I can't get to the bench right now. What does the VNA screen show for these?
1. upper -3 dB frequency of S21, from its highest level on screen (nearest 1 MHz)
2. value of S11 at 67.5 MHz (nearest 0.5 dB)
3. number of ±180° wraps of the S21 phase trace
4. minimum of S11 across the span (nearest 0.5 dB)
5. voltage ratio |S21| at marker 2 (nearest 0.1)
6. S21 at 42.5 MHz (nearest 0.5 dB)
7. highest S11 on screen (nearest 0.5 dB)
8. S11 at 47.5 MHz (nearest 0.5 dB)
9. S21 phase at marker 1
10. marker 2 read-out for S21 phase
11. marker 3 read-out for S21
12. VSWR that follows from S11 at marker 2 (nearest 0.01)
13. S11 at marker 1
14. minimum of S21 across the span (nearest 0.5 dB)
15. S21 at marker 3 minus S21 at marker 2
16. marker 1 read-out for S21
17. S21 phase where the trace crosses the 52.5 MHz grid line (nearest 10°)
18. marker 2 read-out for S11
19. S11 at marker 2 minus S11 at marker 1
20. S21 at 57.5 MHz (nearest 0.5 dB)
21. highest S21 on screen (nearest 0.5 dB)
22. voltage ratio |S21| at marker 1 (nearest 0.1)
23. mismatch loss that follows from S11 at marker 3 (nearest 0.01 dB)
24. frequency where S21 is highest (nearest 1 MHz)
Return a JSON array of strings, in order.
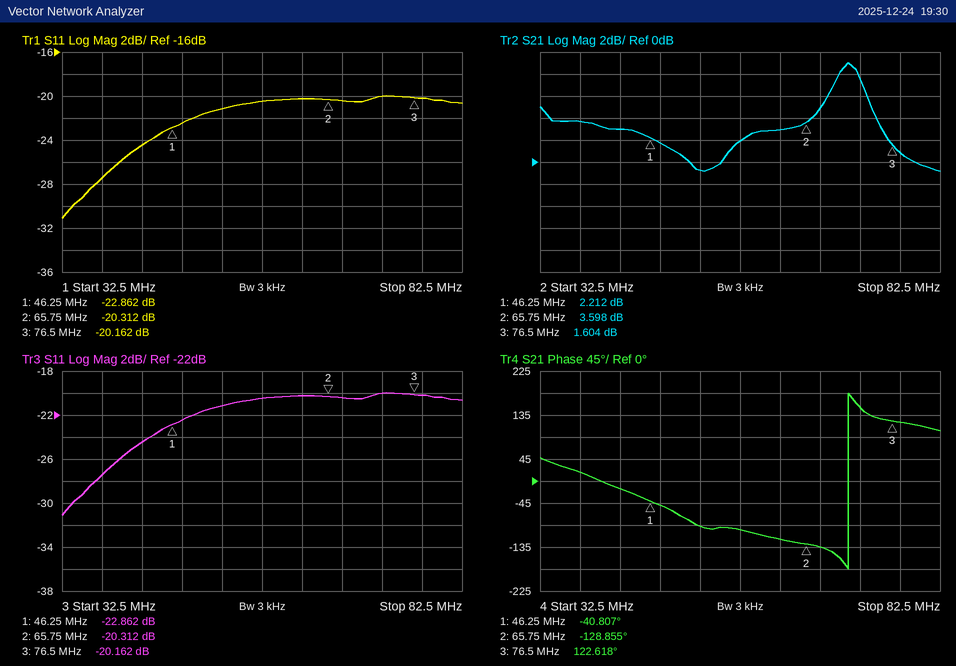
["73 MHz", "-20.5 dB", "1", "-31.0 dB", "1.5", "3.0 dB", "-20.0 dB", "-22.5 dB", "-40.807°", "-128.855°", "1.604 dB", "1.21", "-22.862 dB", "-1.0 dB", "-1.994 dB", "2.212 dB", "-90°", "-20.312 dB", "2.550 dB", "2.0 dB", "9.0 dB", "1.3", "0.04 dB", "71 MHz"]
